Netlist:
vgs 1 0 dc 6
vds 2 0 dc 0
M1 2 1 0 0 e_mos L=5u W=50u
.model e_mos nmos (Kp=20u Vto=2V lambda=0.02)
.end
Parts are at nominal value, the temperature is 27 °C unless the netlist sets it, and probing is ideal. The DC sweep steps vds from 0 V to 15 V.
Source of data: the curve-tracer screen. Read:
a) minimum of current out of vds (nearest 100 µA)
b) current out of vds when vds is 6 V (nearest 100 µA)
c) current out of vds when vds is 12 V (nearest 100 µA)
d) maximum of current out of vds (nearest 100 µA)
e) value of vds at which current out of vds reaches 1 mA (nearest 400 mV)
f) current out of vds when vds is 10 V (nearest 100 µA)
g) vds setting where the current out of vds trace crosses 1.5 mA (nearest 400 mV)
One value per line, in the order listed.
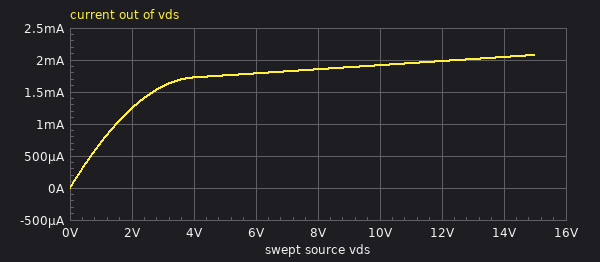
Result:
0 A
1.8 mA
2.0 mA
2.1 mA
1.6 V
1.9 mA
2.8 V
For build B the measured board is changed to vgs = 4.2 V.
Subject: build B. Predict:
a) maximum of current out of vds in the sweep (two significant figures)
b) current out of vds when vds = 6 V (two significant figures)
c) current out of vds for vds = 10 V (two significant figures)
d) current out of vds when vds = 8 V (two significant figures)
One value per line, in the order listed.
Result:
630 µA
540 µA
580 µA
560 µA
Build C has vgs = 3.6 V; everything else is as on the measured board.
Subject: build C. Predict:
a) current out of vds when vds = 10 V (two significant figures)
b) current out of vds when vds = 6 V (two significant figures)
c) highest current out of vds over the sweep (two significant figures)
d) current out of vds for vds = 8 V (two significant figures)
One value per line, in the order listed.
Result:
310 µA
290 µA
330 µA
300 µA
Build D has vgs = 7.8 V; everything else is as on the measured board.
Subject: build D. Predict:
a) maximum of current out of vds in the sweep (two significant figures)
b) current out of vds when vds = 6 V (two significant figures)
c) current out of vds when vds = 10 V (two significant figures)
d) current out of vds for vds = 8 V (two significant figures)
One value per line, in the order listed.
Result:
4.4 mA
3.8 mA
4.0 mA
3.9 mA
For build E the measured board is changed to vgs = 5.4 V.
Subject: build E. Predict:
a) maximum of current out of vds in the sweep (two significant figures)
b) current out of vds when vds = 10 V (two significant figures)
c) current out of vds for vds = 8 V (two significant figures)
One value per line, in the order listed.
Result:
1.5 mA
1.4 mA
1.3 mA
